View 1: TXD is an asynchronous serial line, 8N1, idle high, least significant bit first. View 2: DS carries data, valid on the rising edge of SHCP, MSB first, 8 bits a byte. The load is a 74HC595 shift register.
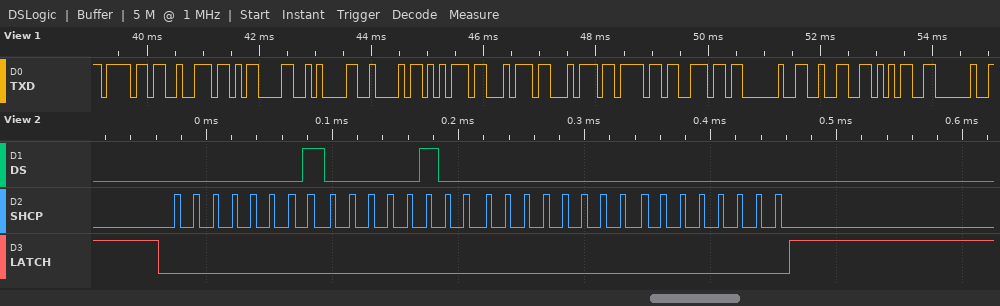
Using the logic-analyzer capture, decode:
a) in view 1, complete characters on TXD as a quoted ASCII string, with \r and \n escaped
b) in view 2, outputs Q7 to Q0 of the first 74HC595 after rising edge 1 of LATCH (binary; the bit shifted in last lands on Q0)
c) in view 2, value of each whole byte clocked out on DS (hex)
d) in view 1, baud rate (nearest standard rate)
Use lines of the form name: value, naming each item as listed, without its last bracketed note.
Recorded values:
in view 1, complete characters on TXD as a quoted ASCII string, with \r and \n escaped: "or\r\nButton 25 "
in view 2, outputs Q7 to Q0 of the first 74HC595 after rising edge 1 of LATCH: 00000000
in view 2, value of each whole byte clocked out on DS: 01 04 00 00
in view 1, baud rate: 9600 baud
